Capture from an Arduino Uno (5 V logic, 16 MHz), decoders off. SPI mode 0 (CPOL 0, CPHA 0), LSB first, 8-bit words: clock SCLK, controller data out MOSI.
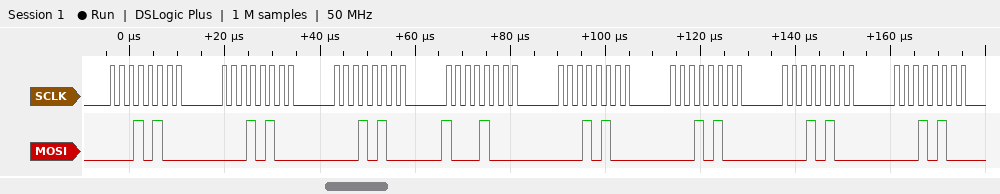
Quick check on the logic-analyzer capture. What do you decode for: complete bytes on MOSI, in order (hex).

28 28 28 11 28 28 28 28
